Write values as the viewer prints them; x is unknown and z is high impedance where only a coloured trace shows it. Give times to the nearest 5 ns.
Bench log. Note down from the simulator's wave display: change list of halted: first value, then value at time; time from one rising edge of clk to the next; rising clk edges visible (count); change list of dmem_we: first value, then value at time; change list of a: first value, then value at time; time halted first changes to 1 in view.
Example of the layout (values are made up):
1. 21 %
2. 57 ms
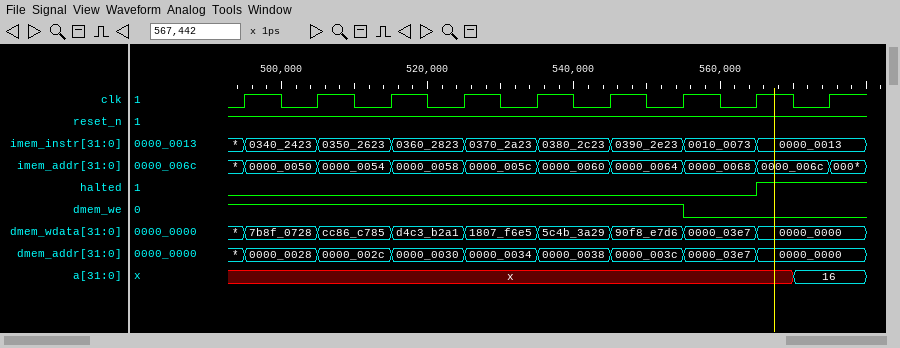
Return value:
1. 0, 1 at 565 ns
2. 10 ns
3. 9
4. 1, 0 at 555 ns
5. x, 16 at 570 ns
6. 565 ns
